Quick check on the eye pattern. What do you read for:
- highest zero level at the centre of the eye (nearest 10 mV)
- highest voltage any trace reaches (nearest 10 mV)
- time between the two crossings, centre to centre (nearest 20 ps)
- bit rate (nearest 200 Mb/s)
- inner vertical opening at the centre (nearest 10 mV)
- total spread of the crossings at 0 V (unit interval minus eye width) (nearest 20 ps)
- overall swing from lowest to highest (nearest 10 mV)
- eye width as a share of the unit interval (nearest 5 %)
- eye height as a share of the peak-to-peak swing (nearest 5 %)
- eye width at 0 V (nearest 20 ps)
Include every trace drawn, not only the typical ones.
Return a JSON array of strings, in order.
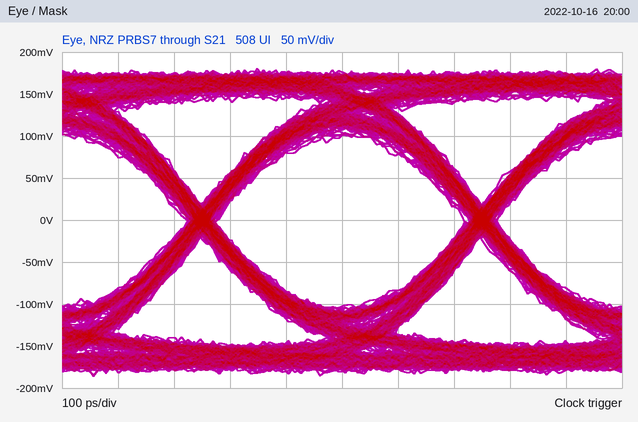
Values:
["-100 mV", "180 mV", "500 ps", "2.0 Gb/s", "200 mV", "60 ps", "370 mV", "90 %", "55 %", "440 ps"]
